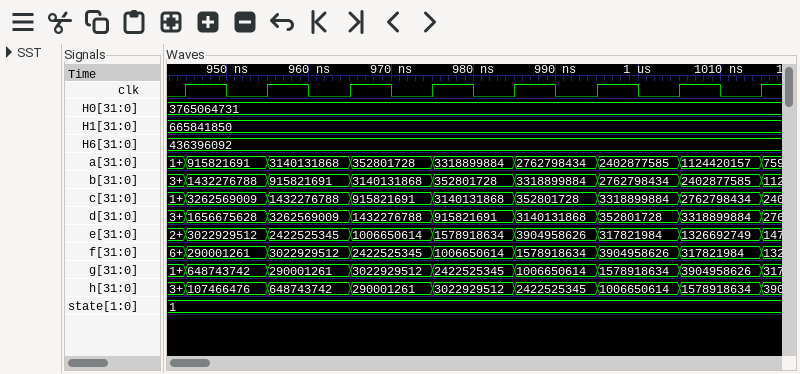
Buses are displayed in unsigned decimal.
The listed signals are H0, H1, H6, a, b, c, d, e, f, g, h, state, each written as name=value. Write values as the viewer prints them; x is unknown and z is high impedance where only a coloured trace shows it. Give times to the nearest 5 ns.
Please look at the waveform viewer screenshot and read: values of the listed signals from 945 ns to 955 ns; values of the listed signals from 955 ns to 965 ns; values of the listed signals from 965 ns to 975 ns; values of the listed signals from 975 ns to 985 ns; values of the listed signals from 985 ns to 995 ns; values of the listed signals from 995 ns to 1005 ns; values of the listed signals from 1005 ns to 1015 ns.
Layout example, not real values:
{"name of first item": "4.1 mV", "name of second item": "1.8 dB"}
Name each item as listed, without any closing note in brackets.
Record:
{"values of the listed signals from 945 ns to 955 ns": "H0=3765064731, H1=665841850, H6=436396092, a=915821691, b=1432276788, c=3262569009, d=1656675628, e=3022929512, f=290001261, g=648743742, h=107466476, state=1", "values of the listed signals from 955 ns to 965 ns": "H0=3765064731, H1=665841850, H6=436396092, a=3140131868, b=915821691, c=1432276788, d=3262569009, e=2422525345, f=3022929512, g=290001261, h=648743742, state=1", "values of the listed signals from 965 ns to 975 ns": "H0=3765064731, H1=665841850, H6=436396092, a=352801728, b=3140131868, c=915821691, d=1432276788, e=1006650614, f=2422525345, g=3022929512, h=290001261, state=1", "values of the listed signals from 975 ns to 985 ns": "H0=3765064731, H1=665841850, H6=436396092, a=3318899884, b=352801728, c=3140131868, d=915821691, e=1578918634, f=1006650614, g=2422525345, h=3022929512, state=1", "values of the listed signals from 985 ns to 995 ns": "H0=3765064731, H1=665841850, H6=436396092, a=2762798434, b=3318899884, c=352801728, d=3140131868, e=3904958626, f=1578918634, g=1006650614, h=2422525345, state=1", "values of the listed signals from 995 ns to 1005 ns": "H0=3765064731, H1=665841850, H6=436396092, a=2402877585, b=2762798434, c=3318899884, d=352801728, e=317821984, f=3904958626, g=1578918634, h=1006650614, state=1", "values of the listed signals from 1005 ns to 1015 ns": "H0=3765064731, H1=665841850, H6=436396092, a=1124420157, b=2402877585, c=2762798434, d=3318899884, e=1326692749, f=317821984, g=3904958626, h=1578918634, state=1"}
